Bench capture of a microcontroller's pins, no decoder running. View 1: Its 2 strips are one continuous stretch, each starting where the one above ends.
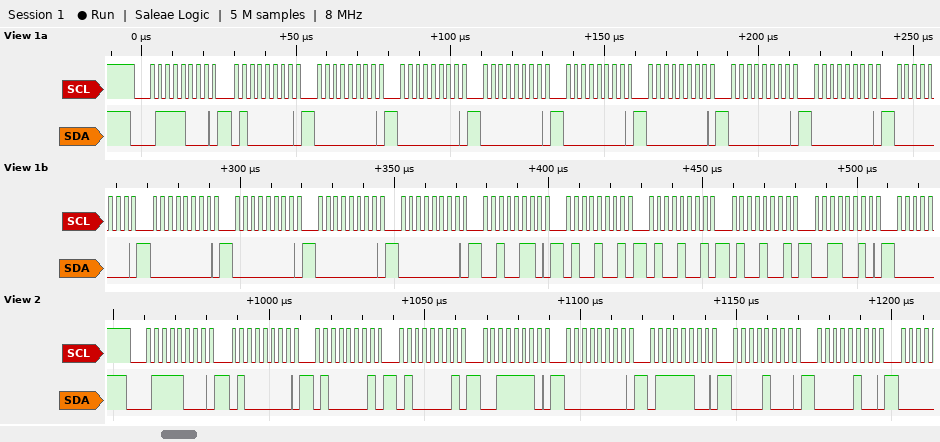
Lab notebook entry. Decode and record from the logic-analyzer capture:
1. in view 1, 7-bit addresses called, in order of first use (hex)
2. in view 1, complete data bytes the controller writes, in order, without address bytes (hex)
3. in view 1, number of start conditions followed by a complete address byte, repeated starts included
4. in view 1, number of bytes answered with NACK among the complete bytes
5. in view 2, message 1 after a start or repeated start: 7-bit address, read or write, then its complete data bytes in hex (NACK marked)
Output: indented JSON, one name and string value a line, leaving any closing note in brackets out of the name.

{
  "in view 1, 7-bit addresses called, in order of first use": "0x3C",
  "in view 1, complete data bytes the controller writes, in order, without address bytes": "40 00 00 00 00 00 00 00 00 00 00 00 00 26 49 49 49 32",
  "in view 1, number of start conditions followed by a complete address byte, repeated starts included": "1",
  "in view 1, number of bytes answered with NACK among the complete bytes": "0",
  "in view 2, message 1 after a start or repeated start: 7-bit address, read or write, then its complete data bytes in hex": "0x3C write: 40 41 41 3E 00 7C 08 04"
}
